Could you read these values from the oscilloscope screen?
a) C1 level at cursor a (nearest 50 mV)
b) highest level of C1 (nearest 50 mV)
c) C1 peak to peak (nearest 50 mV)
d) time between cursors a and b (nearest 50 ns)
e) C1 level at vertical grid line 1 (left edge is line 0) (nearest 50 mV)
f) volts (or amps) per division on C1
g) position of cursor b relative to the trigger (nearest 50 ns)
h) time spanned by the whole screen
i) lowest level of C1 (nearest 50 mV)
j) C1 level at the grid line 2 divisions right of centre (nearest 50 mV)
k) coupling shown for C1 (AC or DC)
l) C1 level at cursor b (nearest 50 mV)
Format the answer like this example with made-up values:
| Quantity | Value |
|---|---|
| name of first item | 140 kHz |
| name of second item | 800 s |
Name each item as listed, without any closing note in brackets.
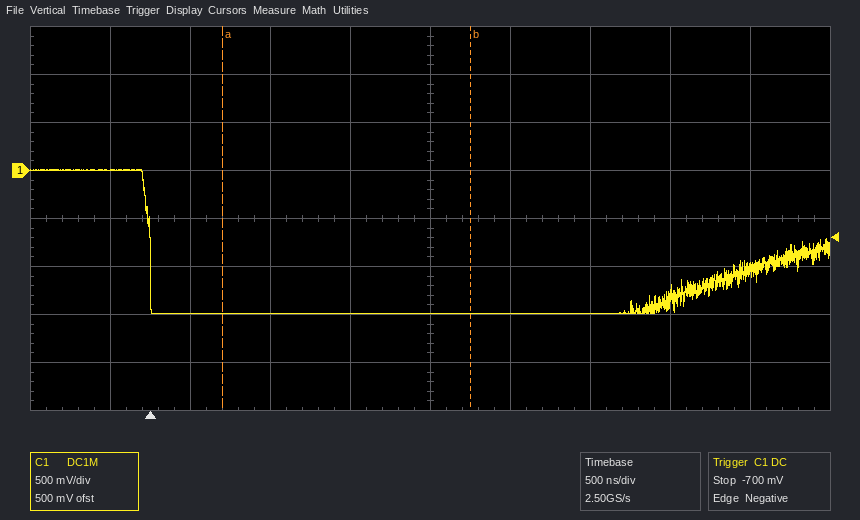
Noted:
| Quantity | Value |
|---|---|
| C1 level at cursor a | -1.50 V |
| highest level of C1 | 0 mV |
| C1 peak to peak | 1.50 V |
| time between cursors a and b | 1.55 µs |
| C1 level at vertical grid line 1 (left edge is line 0) | 0 mV |
| volts (or amps) per division on C1 | 500 mV |
| position of cursor b relative to the trigger | +2.00 µs |
| time spanned by the whole screen | 5 µs |
| lowest level of C1 | -1.50 V |
| C1 level at the grid line 2 divisions right of centre | -1.50 V |
| coupling shown for C1 | DC |
| C1 level at cursor b | -1.50 V |
